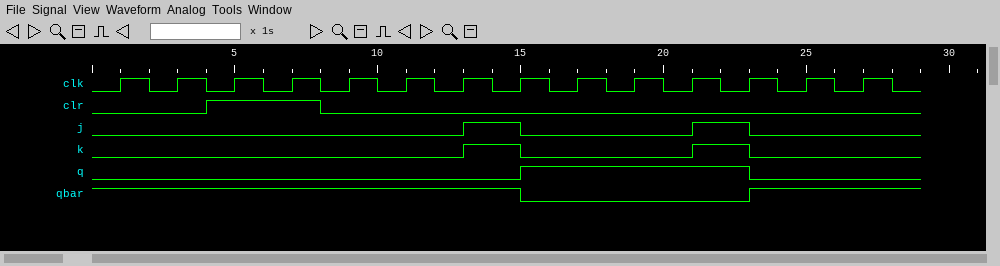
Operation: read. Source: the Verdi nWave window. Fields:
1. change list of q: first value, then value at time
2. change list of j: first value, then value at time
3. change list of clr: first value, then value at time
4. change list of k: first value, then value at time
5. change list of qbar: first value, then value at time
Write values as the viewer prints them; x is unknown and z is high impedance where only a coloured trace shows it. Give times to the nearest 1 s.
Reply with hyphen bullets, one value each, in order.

- 0, 1 at 15 s, 0 at 23 s
- 0, 1 at 13 s, 0 at 15 s, 1 at 21 s, 0 at 23 s
- 0, 1 at 4 s, 0 at 8 s
- 0, 1 at 13 s, 0 at 15 s, 1 at 21 s, 0 at 23 s
- 1, 0 at 15 s, 1 at 23 s
